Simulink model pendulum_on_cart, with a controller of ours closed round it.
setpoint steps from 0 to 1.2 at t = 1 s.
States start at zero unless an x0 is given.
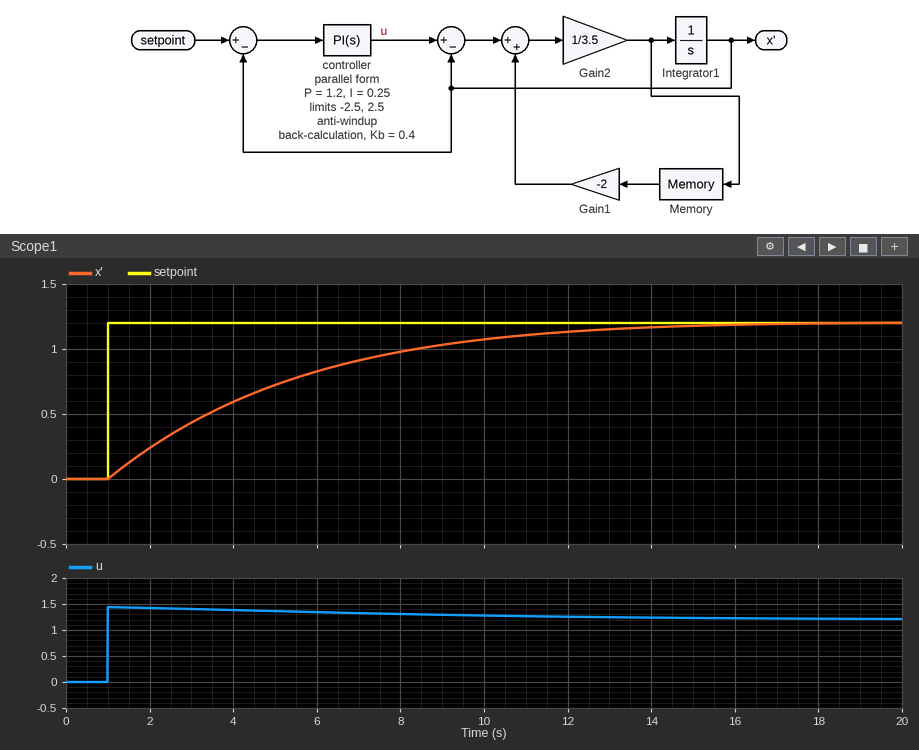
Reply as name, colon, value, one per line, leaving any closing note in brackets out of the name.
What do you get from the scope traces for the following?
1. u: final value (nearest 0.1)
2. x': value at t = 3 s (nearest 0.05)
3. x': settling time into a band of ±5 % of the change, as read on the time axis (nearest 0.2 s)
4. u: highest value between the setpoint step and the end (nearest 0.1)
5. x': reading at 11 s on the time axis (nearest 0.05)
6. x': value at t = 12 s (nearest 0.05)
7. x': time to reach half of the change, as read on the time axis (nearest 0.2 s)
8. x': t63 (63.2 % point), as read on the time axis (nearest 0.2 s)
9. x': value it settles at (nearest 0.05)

u: final value: 1.2
x': value at t = 3 s: 0.45
x': settling time into a band of ±5 % of the change, as read on the time axis: 12.4 s
u: highest value between the setpoint step and the end: 1.4
x': reading at 11 s on the time axis: 1.10
x': value at t = 12 s: 1.15
x': time to reach half of the change, as read on the time axis: 4.0 s
x': t63 (63.2 % point), as read on the time axis: 5.4 s
x': value it settles at: 1.20
